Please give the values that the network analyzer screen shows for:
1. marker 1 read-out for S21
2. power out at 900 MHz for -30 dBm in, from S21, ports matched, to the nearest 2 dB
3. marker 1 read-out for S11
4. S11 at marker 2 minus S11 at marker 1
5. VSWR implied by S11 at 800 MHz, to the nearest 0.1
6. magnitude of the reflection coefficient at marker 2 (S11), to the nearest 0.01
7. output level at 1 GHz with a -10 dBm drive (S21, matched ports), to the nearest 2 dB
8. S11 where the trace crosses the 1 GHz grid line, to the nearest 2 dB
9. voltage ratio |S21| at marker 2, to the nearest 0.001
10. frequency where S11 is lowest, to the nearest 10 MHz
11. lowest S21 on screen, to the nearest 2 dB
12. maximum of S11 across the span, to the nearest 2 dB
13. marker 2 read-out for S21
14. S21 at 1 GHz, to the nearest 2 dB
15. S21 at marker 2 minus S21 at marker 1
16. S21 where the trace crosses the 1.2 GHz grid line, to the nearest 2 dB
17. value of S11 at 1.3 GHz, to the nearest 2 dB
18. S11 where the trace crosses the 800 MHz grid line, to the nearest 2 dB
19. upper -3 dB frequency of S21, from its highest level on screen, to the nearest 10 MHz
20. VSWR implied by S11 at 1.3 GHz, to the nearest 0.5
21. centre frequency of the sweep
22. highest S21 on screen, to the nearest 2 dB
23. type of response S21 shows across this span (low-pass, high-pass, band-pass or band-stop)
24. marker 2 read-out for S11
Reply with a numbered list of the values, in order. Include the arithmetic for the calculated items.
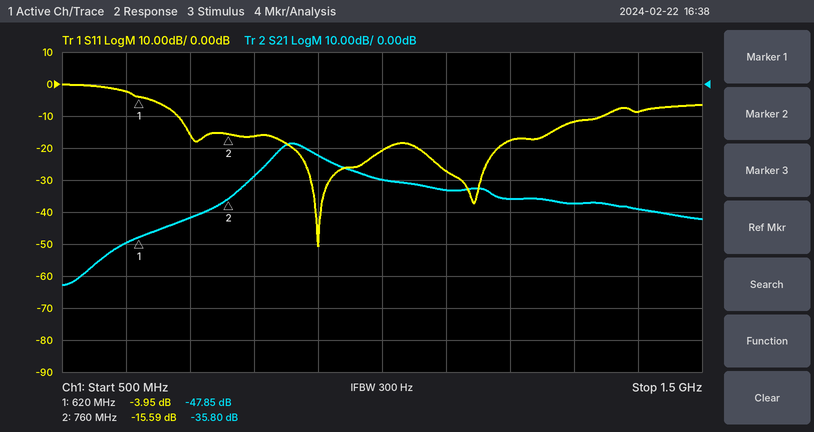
1. -47.85 dB
2. -30 dBm + (-22 dB) = -52 dBm
3. -3.95 dB
4. -15.59 − (-3.95) = -11.64 dB
5. |Γ| = 10^(-16/20) = 0.1585; VSWR = (1 + 0.1585)/(1 − 0.1585) ≈ 1.4
6. 10^(-15.59/20) ≈ 0.17
7. -10 dBm + (-30 dB) = -40 dBm
8. -20 dB
9. 10^(-35.8/20) ≈ 0.016
10. 900 MHz
11. -62 dB
12. 0 dB
13. -35.80 dB
14. -30 dB
15. -35.8 − (-47.85) = 12.05 dB
16. -36 dB
17. -12 dB
18. -16 dB
19. 890 MHz
20. |Γ| = 10^(-12/20) = 0.2512; VSWR = (1 + 0.2512)/(1 − 0.2512) ≈ 1.67, so 1.5 to the nearest 0.5
21. 1 GHz
22. -18 dB
23. band-pass
24. -15.59 dB
